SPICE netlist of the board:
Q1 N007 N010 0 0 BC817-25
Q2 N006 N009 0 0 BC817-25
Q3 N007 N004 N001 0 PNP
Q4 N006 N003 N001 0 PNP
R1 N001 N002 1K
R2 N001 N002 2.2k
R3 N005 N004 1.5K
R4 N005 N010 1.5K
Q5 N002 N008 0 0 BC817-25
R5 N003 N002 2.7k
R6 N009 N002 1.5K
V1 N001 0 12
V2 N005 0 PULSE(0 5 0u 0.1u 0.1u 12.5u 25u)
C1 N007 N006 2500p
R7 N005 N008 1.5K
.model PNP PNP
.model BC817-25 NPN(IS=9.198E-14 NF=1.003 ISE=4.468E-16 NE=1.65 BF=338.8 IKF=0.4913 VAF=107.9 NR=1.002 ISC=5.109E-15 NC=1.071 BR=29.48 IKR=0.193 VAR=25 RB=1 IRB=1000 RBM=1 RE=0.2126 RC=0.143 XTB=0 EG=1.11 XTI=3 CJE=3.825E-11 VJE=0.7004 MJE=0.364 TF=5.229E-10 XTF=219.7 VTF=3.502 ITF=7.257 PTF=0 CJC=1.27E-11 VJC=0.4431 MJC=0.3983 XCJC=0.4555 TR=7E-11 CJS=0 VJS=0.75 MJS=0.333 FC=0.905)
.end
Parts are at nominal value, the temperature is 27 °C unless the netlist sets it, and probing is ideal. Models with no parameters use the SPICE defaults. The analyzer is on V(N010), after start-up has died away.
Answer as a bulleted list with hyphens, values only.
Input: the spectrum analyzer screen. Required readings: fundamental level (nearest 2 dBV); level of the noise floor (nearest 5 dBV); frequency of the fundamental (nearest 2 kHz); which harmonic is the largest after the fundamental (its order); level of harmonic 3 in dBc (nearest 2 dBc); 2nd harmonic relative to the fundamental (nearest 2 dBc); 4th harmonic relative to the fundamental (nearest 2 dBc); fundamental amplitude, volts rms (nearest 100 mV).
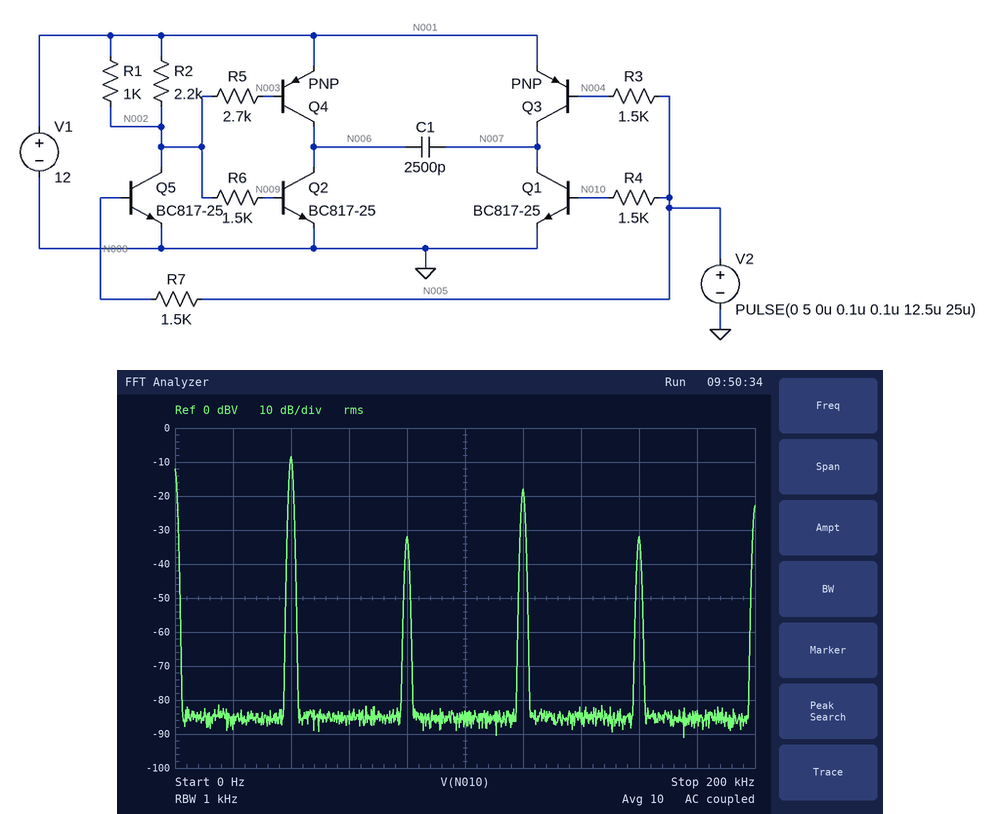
- -8 dBV
- -85 dBV
- 40 kHz
- 3
- -10 dBc
- -24 dBc
- -24 dBc
- 400 mV
